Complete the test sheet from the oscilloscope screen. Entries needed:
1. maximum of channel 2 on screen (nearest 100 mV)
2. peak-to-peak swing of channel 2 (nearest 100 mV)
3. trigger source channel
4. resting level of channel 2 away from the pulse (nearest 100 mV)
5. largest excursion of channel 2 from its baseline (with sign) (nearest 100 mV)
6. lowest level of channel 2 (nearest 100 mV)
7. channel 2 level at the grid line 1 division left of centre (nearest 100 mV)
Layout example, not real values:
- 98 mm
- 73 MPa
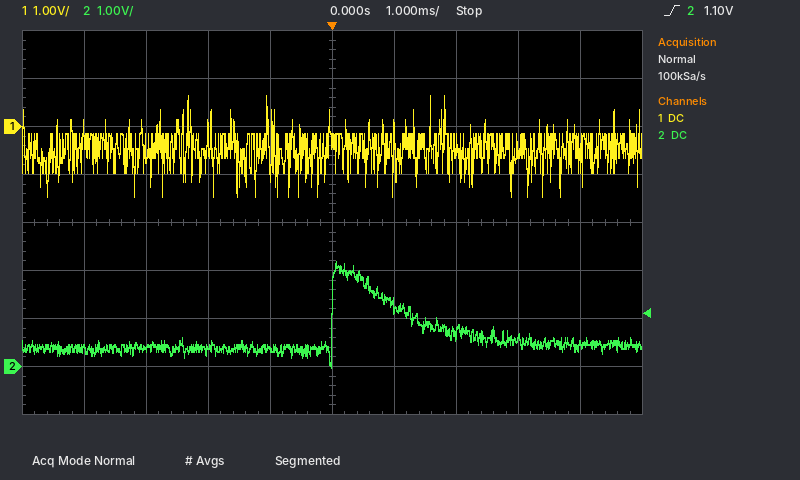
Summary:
- 2.2 V
- 2.2 V
- channel 2
- 400 mV
- +1.8 V
- 0.0 V
- 400 mV
